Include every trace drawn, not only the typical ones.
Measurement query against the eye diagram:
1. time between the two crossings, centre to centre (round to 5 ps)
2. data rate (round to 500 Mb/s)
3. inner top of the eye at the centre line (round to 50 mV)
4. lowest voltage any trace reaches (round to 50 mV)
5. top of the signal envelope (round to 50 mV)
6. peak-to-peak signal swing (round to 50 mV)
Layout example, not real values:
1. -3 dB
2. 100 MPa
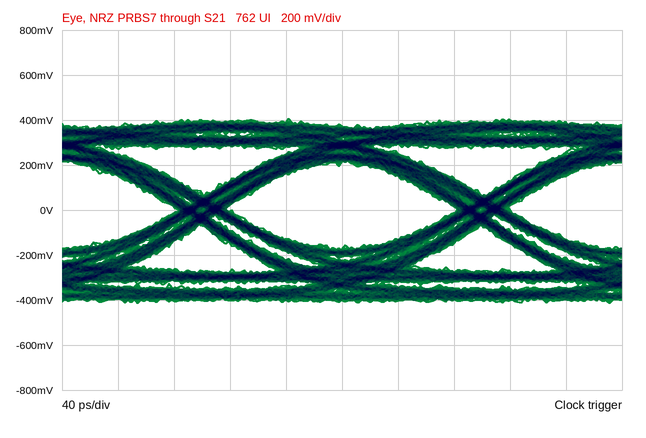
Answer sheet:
1. 200 ps
2. 5.0 Gb/s
3. 200 mV
4. -400 mV
5. 400 mV
6. 800 mV
